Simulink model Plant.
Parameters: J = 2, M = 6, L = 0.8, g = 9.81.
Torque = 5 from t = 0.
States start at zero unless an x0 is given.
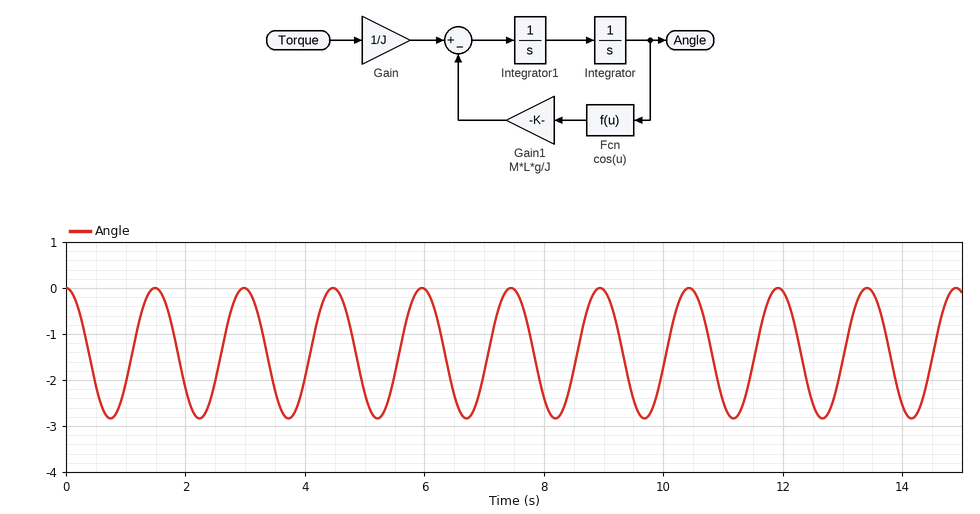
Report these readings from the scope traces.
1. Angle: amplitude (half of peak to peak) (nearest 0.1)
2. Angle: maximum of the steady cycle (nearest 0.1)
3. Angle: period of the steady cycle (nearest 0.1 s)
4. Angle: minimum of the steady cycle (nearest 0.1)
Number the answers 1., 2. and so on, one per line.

1. 1.4
2. 0.0
3. 1.5 s
4. -2.8
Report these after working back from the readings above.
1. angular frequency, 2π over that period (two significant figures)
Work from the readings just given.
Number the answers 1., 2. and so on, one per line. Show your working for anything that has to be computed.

1. 2π / 1.5 = 4.2 rad/s
